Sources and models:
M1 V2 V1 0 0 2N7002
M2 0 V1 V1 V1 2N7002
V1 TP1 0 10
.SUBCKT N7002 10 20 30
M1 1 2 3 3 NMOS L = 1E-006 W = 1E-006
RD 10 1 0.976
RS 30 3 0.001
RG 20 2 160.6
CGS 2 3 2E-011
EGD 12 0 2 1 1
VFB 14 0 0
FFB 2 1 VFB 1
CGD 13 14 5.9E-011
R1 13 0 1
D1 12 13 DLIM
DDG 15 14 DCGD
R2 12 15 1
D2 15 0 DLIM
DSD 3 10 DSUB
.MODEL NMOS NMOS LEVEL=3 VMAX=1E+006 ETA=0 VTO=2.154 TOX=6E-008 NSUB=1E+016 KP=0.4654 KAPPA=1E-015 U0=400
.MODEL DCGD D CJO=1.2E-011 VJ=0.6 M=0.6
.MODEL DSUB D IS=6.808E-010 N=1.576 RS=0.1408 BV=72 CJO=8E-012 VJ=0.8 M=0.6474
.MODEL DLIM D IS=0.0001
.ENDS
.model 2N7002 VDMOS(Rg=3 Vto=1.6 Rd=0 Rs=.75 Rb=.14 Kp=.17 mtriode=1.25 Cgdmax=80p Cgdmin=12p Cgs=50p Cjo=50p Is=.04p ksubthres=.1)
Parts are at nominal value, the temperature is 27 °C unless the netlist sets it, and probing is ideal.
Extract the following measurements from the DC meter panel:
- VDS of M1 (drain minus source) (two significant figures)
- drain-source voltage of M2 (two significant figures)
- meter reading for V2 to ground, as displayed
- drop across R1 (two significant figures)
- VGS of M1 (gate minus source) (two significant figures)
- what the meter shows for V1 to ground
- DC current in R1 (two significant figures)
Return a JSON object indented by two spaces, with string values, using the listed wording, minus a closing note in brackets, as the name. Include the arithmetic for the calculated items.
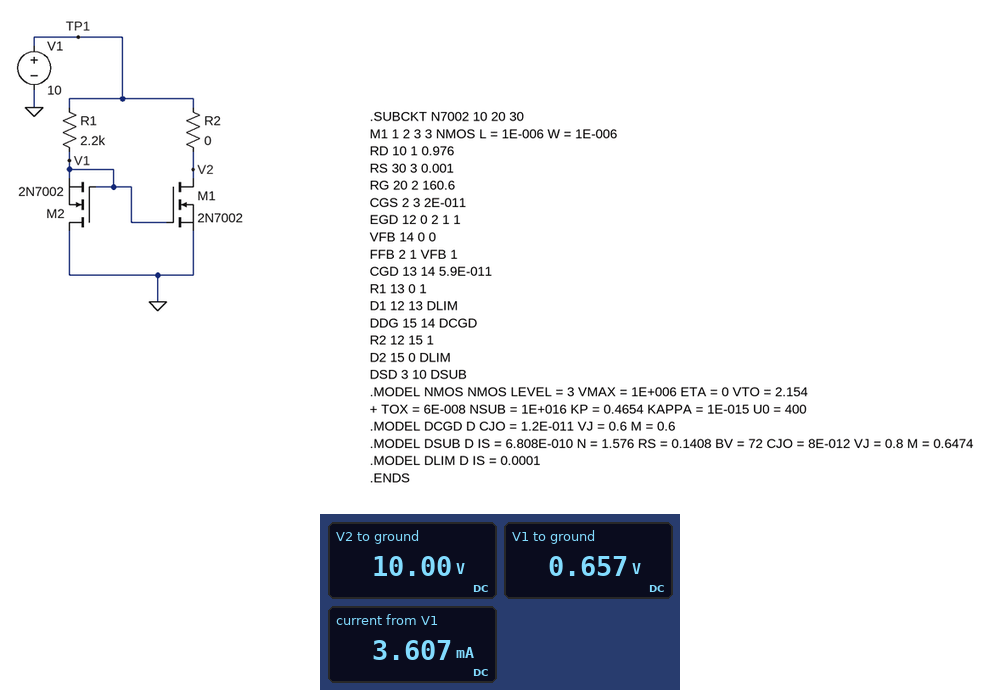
{
  "VDS of M1 (drain minus source)": "10 V = 10 V",
  "drain-source voltage of M2": "0 V - 657 mV = -660 mV",
  "meter reading for V2 to ground, as displayed": "10.00 V",
  "drop across R1": "10 V - 657 mV = 9.3 V",
  "VGS of M1 (gate minus source)": "657 mV = 660 mV",
  "what the meter shows for V1 to ground": "0.657 V",
  "DC current in R1": "(10 V - 657 mV) / 2.2 kΩ = 4.2 mA"
}
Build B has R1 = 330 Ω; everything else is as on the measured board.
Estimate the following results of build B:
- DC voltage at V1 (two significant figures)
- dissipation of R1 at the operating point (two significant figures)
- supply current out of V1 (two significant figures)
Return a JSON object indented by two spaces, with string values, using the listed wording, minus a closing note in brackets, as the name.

{
  "DC voltage at V1": "710 mV",
  "dissipation of R1 at the operating point": "260 mW",
  "supply current out of V1": "29 mA"
}
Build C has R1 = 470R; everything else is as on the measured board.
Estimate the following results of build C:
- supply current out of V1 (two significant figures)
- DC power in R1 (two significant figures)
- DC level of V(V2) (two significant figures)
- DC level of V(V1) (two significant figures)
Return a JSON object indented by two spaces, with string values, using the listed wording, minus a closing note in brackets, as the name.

{
  "supply current out of V1": "20 mA",
  "DC power in R1": "180 mW",
  "DC level of V(V2)": "10 V",
  "DC level of V(V1)": "700 mV"
}
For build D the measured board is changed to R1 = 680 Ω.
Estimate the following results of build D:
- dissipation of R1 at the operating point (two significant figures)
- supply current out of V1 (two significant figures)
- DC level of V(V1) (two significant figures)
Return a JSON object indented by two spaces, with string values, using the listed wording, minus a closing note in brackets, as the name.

{
  "dissipation of R1 at the operating point": "130 mW",
  "supply current out of V1": "15 mA",
  "DC level of V(V1)": "690 mV"
}
